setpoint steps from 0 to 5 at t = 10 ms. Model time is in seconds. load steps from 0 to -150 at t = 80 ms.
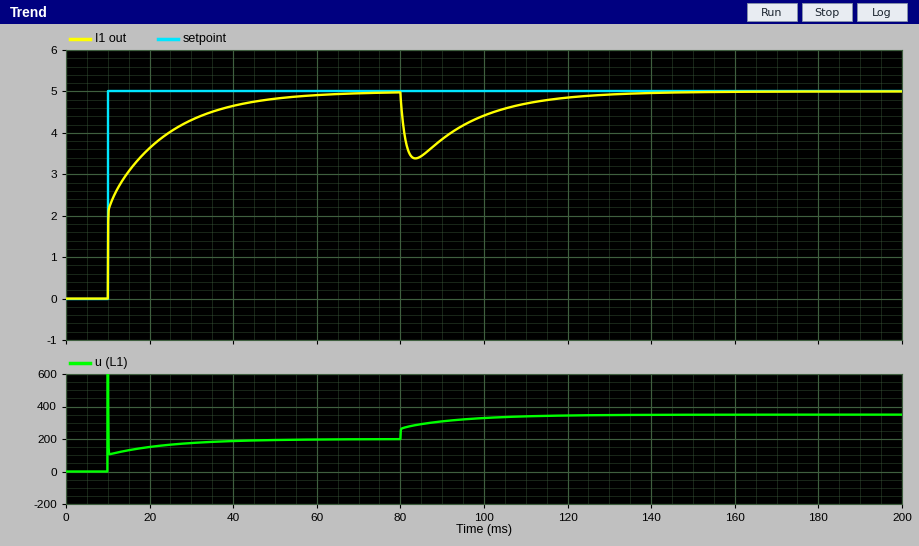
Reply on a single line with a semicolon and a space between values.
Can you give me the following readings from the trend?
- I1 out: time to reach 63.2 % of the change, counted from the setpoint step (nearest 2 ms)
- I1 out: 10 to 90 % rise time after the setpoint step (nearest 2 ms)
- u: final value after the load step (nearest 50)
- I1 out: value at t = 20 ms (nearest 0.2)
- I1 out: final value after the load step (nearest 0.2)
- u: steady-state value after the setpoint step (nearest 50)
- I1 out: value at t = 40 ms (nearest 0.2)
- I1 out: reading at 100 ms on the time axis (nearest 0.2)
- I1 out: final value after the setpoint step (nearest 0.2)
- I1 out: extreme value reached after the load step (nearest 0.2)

6 ms; 24 ms; 350; 3.6; 5.0; 200; 4.6; 4.4; 5.0; 3.4
